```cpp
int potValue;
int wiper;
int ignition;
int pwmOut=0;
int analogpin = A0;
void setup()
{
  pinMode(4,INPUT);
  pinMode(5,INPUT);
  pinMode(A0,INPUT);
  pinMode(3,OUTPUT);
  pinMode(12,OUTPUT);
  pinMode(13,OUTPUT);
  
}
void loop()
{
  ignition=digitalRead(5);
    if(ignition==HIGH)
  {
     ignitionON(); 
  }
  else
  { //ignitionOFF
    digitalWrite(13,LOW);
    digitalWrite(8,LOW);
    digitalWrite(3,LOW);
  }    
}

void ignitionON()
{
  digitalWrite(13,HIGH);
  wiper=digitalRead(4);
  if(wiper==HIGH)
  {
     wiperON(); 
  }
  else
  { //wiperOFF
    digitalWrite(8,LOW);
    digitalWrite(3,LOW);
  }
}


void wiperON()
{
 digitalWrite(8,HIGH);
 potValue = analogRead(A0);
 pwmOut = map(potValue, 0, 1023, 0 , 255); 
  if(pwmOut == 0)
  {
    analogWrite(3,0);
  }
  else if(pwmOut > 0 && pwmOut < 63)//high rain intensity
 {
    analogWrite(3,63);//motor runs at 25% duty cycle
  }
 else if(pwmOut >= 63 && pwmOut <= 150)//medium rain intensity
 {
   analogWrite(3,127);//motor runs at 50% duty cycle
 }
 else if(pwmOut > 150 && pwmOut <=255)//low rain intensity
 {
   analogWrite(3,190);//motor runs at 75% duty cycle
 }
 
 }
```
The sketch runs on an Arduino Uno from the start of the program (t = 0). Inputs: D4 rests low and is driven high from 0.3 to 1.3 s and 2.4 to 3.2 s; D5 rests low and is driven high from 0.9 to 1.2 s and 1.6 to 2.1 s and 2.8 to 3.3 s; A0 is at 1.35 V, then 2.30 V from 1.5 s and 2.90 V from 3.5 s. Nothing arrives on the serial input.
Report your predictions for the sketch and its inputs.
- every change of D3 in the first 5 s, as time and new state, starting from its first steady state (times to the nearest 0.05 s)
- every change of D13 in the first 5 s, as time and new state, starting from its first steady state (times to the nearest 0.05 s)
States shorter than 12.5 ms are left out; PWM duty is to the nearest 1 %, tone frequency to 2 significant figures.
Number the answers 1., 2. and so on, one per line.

1. 0 s low; 0.9 s PWM 50 %; 1.2 s low; 2.8 s PWM 50 %; 3.2 s low
2. 0 s low; 0.9 s high; 1.2 s low; 1.6 s high; 2.1 s low; 2.8 s high; 3.3 s low
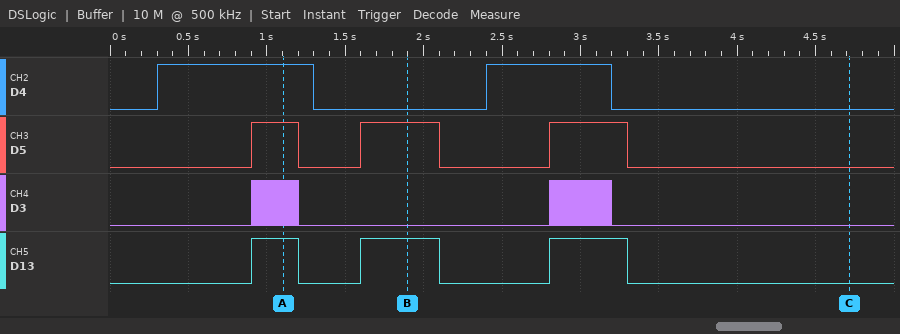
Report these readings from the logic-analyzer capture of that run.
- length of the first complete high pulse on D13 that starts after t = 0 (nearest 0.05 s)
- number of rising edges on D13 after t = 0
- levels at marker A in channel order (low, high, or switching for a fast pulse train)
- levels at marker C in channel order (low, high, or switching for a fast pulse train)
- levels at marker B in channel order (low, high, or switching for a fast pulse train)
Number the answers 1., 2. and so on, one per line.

1. 0.30 s
2. 3
3. D4 high, D5 high, D3 switching, D13 high
4. D4 low, D5 low, D3 low, D13 low
5. D4 low, D5 high, D3 low, D13 high
